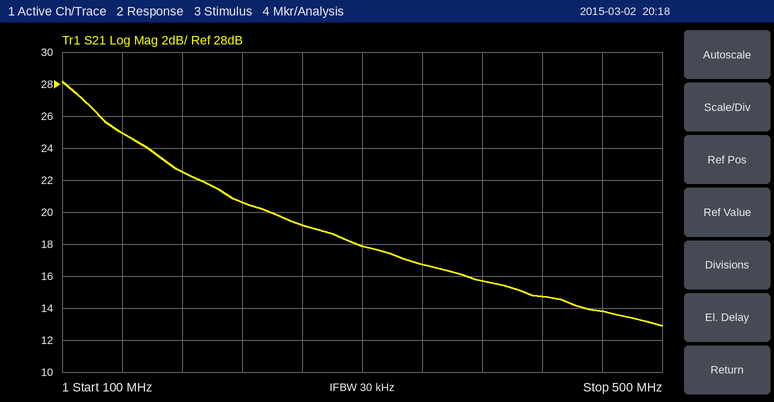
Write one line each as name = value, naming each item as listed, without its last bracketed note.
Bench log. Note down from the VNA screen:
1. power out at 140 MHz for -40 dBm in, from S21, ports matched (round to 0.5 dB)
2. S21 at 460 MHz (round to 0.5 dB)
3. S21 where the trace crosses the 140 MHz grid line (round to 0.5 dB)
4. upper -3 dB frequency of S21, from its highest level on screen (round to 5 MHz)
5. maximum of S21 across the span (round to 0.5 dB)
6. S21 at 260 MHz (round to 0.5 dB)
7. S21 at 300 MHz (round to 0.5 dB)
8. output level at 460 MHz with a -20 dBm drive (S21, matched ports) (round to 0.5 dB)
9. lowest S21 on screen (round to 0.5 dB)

power out at 140 MHz for -40 dBm in, from S21, ports matched = -15.0 dBm
S21 at 460 MHz = 14.0 dB
S21 where the trace crosses the 140 MHz grid line = 25.0 dB
upper -3 dB frequency of S21, from its highest level on screen = 135 MHz
maximum of S21 across the span = 28.0 dB
S21 at 260 MHz = 19.0 dB
S21 at 300 MHz = 18.0 dB
output level at 460 MHz with a -20 dBm drive (S21, matched ports) = -6.0 dBm
lowest S21 on screen = 13.0 dB
